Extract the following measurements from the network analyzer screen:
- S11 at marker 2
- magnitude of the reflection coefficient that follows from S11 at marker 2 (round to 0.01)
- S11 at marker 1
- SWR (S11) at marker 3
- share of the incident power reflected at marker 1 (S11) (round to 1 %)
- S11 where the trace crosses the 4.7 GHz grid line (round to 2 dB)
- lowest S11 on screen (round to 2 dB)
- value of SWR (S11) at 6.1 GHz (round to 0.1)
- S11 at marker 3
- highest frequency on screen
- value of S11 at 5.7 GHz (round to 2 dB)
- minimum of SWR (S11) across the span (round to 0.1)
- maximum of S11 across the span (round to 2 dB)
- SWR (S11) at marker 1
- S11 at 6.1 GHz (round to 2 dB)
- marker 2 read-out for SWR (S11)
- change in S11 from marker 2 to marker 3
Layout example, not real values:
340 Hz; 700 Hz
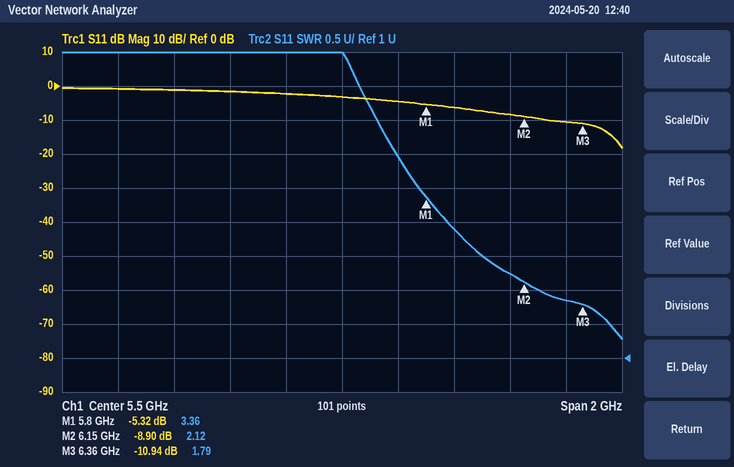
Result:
-8.90 dB; 0.36; -5.32 dB; 1.79; 29 %; 0 dB; -18 dB; 2.2; -10.94 dB; 6.5 GHz; -4 dB; 1.3; 0 dB; 3.36; -8 dB; 2.12; -2.04 dB
